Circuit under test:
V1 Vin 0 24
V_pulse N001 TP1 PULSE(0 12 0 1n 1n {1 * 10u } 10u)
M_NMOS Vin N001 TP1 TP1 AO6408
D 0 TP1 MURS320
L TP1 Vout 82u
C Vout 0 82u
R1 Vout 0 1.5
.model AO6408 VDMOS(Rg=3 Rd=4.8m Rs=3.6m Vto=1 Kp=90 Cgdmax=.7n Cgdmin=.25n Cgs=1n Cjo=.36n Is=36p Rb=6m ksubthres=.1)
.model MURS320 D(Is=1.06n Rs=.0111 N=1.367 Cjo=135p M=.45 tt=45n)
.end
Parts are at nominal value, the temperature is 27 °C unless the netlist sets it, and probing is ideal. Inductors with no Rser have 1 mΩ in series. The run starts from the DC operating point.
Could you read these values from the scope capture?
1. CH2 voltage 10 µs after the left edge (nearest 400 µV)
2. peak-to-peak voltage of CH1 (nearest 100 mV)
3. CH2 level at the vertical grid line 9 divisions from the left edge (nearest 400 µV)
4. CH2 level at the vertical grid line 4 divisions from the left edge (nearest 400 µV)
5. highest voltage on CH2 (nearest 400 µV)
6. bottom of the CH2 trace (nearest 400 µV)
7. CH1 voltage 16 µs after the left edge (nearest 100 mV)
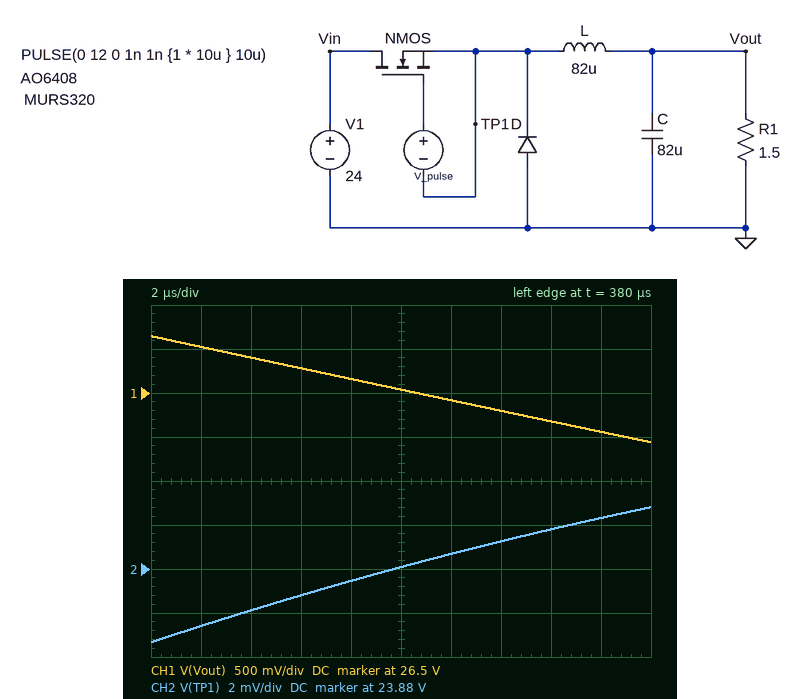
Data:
23.8800 V
1.2 V
23.8824 V
23.8796 V
23.8828 V
23.8768 V
26.2 V
